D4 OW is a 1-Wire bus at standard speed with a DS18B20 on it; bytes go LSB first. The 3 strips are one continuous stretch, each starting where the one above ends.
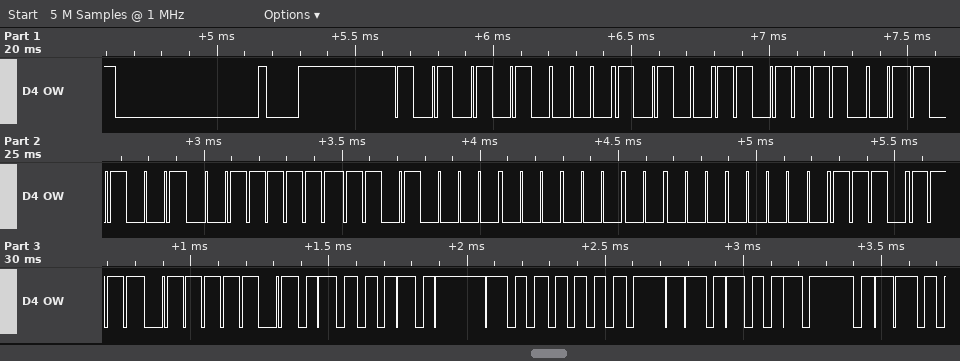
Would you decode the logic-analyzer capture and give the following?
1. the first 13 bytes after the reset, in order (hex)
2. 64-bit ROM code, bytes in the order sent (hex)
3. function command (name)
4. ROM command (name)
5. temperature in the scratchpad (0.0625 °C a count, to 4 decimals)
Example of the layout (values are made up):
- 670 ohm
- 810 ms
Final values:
- 55 28 7B 96 FC 0B 00 00 F7 BE A2 01 4B
- 28 7B 96 FC 0B 00 00 F7
- Read Scratchpad
- Match ROM
- 26.1250 °C
